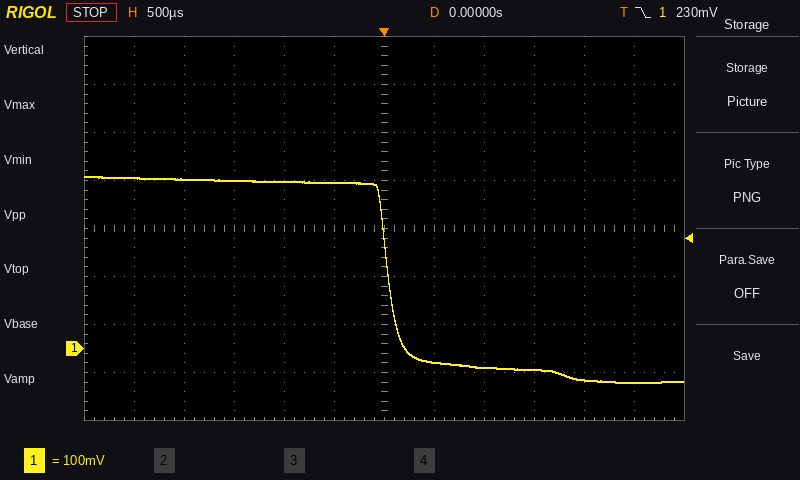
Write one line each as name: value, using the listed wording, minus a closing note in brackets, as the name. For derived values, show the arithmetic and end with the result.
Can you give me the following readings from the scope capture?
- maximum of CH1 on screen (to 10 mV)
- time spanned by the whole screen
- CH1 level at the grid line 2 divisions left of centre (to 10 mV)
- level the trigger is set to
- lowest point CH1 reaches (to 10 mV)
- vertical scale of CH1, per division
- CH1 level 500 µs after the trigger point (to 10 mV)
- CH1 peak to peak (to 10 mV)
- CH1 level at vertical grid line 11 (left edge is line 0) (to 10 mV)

maximum of CH1 on screen: 360 mV
time spanned by the whole screen: 6 ms
CH1 level at the grid line 2 divisions left of centre: 350 mV
level the trigger is set to: 230 mV
lowest point CH1 reaches: -70 mV
vertical scale of CH1, per division: 100 mV
CH1 level 500 µs after the trigger point: -30 mV
CH1 peak to peak: 360 mV − (-70 mV) = 430 mV
CH1 level at vertical grid line 11 (left edge is line 0): -70 mV
